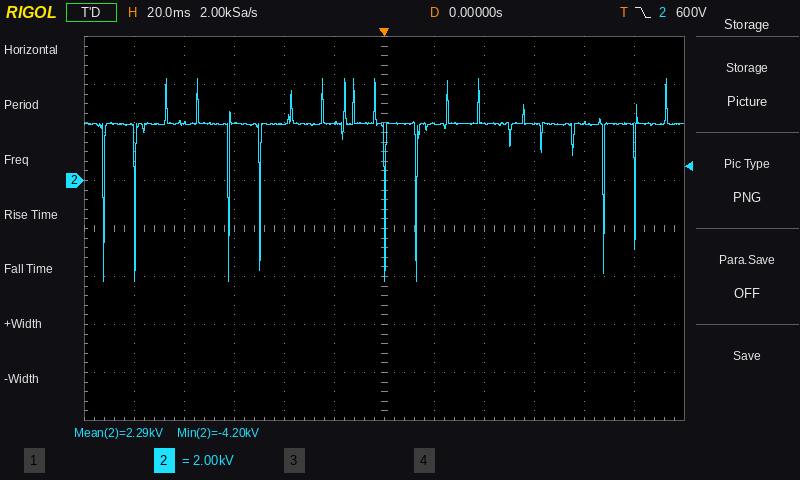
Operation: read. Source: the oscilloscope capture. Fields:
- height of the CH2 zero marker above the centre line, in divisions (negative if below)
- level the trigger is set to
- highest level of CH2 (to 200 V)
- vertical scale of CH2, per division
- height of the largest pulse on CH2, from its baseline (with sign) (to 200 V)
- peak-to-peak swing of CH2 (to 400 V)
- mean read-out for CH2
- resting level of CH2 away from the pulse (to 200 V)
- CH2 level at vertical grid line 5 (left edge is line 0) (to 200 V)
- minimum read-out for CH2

+1.0 div
600 V
4.2 kV
2 kV
-6.6 kV
8.4 kV
2.29 kV
2.4 kV
2.4 kV
-4.20 kV
